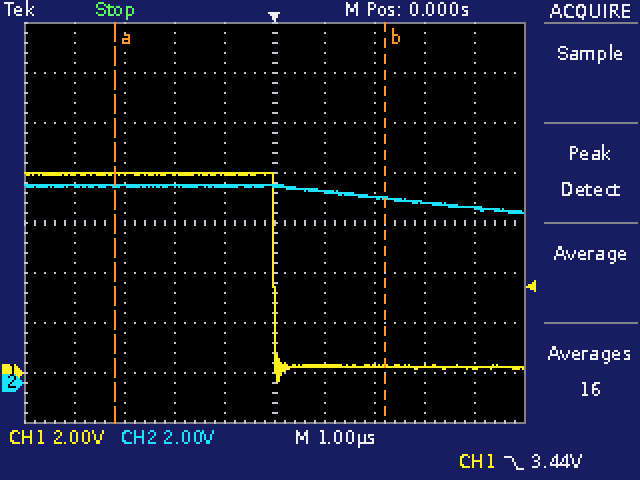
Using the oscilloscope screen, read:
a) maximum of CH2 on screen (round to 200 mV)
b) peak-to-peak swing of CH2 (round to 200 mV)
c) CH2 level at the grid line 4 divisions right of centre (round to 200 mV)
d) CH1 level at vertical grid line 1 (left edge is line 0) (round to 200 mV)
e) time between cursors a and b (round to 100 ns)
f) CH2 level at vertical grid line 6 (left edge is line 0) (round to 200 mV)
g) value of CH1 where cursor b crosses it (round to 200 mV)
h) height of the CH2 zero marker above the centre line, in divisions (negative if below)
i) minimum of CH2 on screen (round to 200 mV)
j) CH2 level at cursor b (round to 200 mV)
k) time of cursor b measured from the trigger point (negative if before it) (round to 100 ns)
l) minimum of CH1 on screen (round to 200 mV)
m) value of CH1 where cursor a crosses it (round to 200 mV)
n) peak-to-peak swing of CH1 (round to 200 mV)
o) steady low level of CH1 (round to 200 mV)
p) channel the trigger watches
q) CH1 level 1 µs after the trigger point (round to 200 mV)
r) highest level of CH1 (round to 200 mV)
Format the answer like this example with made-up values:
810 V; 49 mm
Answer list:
8.0 V; 1.2 V; 7.0 V; 8.0 V; 5.4 µs; 7.6 V; 200 mV; -3.2 div; 6.8 V; 7.4 V; +2.2 µs; -400 mV; 8.0 V; 8.4 V; 200 mV; CH1; 200 mV; 8.0 V
